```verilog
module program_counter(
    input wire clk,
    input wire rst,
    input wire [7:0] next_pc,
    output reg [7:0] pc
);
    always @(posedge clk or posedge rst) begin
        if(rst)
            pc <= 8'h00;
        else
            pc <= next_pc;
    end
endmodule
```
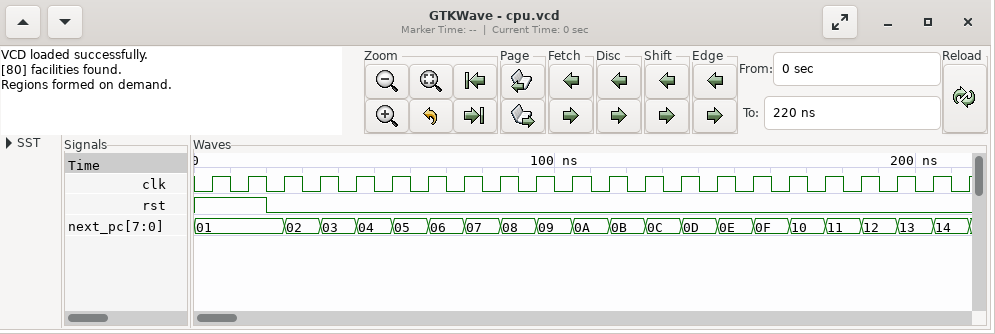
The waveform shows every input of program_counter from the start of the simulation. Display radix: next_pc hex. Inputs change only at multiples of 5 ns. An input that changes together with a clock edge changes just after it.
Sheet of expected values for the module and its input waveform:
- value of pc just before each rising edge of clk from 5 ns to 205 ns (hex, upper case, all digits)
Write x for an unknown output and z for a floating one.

00, 00, 00, 01, 02, 03, 04, 05, 06, 07, 08, 09, 0A, 0B, 0C, 0D, 0E, 0F, 10, 11, 12
